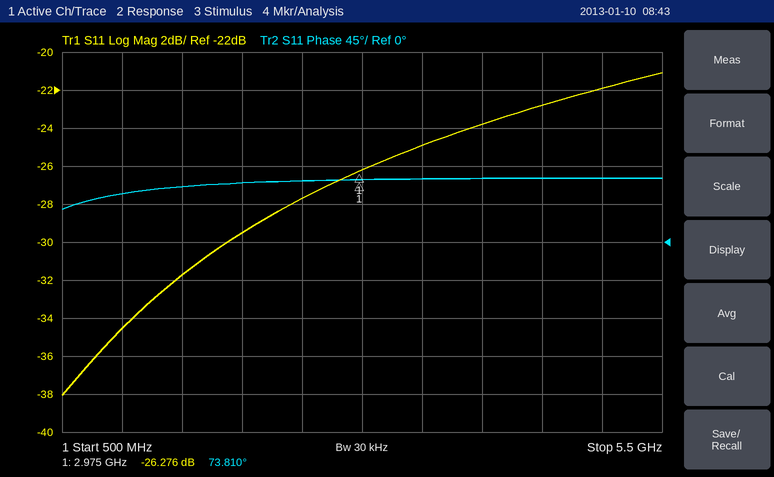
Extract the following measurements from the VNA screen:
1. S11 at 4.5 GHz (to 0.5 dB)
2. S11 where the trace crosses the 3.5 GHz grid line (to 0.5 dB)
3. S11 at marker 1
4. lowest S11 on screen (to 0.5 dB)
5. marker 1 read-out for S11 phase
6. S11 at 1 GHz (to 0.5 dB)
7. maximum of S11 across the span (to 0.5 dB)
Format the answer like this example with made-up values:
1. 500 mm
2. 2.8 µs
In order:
1. -23.0 dB
2. -25.0 dB
3. -26.276 dB
4. -38.0 dB
5. 73.810°
6. -34.5 dB
7. -21.0 dB
